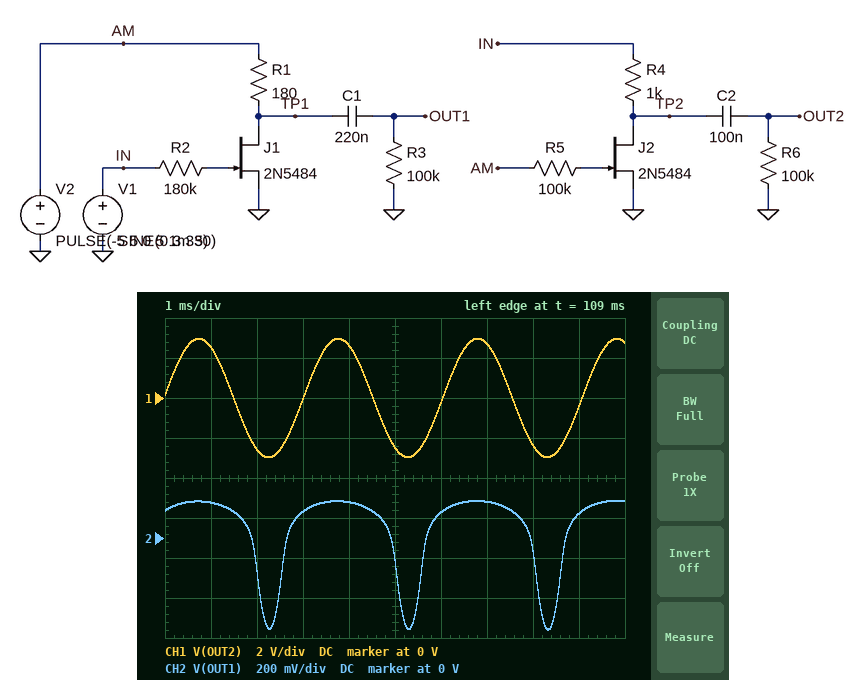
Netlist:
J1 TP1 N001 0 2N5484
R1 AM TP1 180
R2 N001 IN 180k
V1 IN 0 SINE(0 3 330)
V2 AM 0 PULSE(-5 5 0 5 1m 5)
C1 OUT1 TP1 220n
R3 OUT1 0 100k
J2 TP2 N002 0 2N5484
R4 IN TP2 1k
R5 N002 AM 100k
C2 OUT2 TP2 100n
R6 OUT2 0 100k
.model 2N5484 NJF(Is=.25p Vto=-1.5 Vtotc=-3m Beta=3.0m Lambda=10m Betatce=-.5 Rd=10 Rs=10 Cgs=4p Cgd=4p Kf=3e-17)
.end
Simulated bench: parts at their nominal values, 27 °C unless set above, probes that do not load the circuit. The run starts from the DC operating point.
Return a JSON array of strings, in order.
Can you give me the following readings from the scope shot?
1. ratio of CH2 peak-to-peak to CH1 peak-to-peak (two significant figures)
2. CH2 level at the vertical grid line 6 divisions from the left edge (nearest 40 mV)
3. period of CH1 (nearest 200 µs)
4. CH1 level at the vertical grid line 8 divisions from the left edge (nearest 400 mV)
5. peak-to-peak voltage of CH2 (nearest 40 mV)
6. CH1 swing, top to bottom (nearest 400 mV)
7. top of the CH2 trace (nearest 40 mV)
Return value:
["0.11", "120 mV", "3.0 ms", "-2.4 V", "640 mV", "6.0 V", "200 mV"]
